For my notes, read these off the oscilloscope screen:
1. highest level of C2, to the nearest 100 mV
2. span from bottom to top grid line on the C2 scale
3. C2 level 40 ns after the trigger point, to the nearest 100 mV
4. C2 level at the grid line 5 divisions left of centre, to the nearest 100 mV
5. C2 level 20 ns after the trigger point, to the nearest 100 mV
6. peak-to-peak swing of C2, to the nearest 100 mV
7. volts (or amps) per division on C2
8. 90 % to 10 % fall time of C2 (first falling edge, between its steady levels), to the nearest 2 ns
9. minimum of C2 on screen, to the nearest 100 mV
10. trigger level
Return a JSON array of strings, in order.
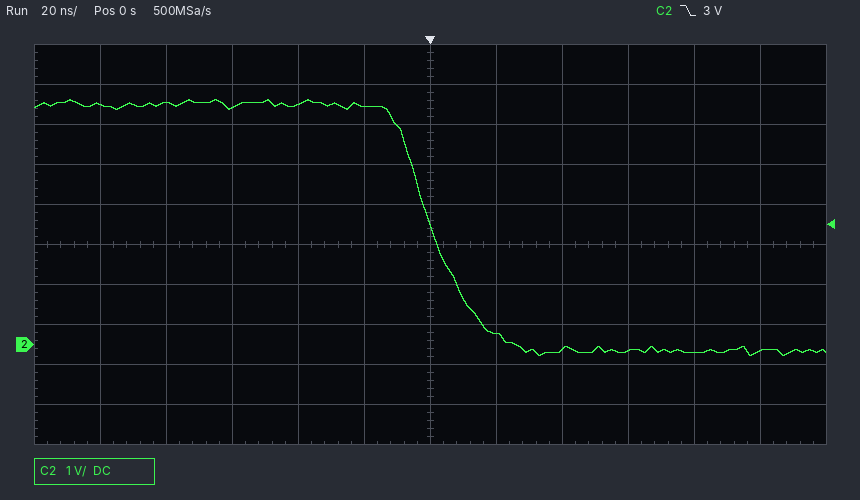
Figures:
["6.1 V", "10 V", "-100 mV", "6.0 V", "300 mV", "6.4 V", "1 V", "26 ns", "-300 mV", "3 V"]
